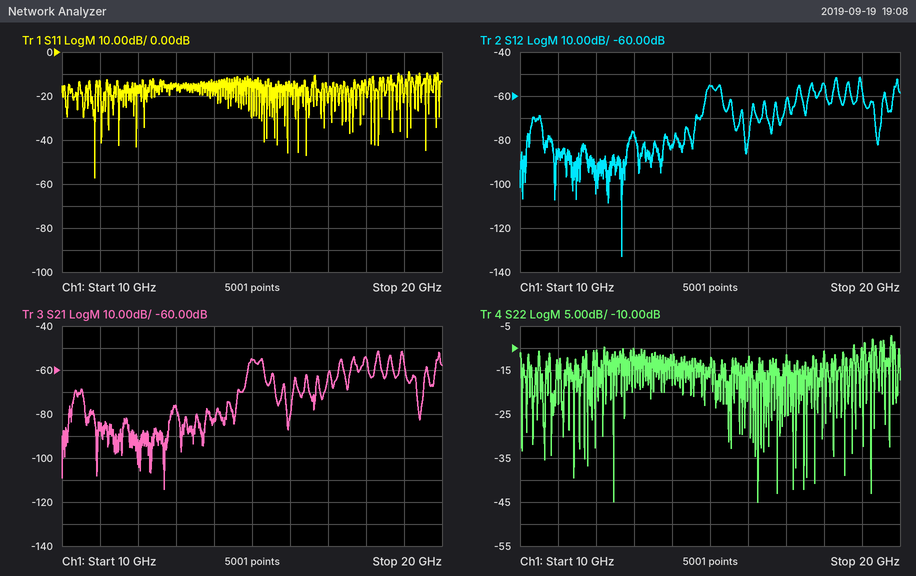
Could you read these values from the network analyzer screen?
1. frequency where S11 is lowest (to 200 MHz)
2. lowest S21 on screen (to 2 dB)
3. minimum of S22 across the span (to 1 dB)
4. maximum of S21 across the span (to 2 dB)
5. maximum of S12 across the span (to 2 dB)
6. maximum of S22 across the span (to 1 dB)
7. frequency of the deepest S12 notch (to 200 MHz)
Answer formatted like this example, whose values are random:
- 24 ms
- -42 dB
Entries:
- 10.8 GHz
- -114 dB
- -45 dB
- -52 dB
- -52 dB
- -7 dB
- 12.6 GHz
